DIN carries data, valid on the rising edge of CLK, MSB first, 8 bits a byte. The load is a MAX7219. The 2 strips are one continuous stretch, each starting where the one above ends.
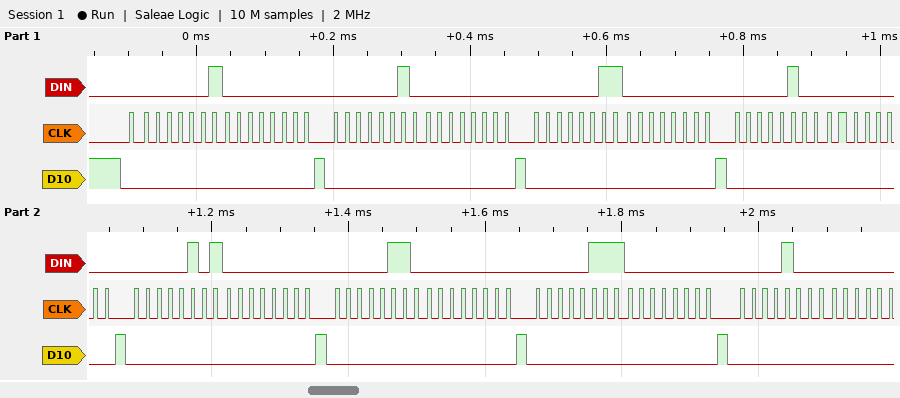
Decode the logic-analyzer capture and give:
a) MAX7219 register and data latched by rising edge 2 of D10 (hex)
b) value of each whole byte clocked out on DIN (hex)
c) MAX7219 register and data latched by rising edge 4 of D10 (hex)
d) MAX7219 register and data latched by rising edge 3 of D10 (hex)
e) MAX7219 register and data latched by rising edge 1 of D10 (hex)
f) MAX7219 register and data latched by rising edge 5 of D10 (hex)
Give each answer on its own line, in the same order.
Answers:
register 0x2, data 0x00
01 00 02 00 03 00 04 00 05 00 06 00 07 00 08
register 0x4, data 0x00
register 0x3, data 0x00
register 0x1, data 0x00
register 0x5, data 0x00
